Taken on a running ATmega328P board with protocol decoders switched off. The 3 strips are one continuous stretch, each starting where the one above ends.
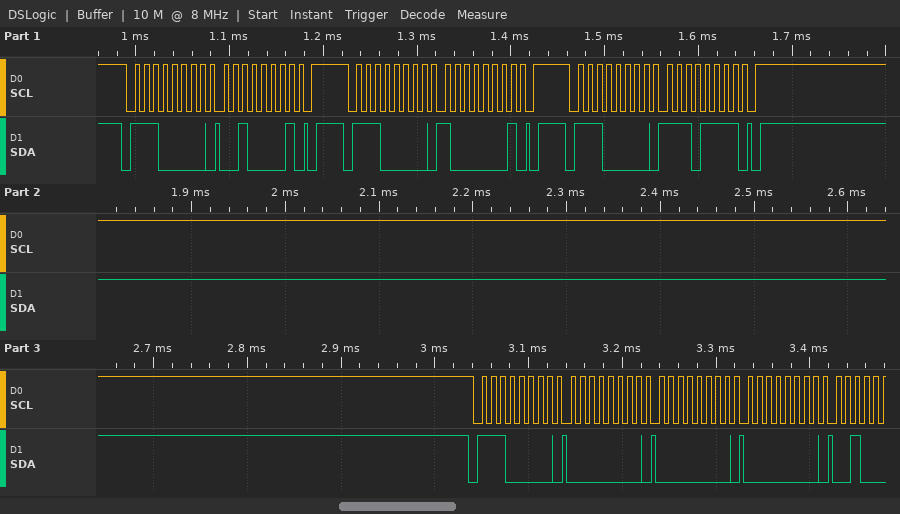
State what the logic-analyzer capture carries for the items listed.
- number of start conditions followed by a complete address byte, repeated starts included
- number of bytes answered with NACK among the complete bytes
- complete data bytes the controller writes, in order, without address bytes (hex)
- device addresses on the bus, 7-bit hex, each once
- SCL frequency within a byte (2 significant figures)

4
0
21 81 EF 00 00 00
0x70
100 kHz
